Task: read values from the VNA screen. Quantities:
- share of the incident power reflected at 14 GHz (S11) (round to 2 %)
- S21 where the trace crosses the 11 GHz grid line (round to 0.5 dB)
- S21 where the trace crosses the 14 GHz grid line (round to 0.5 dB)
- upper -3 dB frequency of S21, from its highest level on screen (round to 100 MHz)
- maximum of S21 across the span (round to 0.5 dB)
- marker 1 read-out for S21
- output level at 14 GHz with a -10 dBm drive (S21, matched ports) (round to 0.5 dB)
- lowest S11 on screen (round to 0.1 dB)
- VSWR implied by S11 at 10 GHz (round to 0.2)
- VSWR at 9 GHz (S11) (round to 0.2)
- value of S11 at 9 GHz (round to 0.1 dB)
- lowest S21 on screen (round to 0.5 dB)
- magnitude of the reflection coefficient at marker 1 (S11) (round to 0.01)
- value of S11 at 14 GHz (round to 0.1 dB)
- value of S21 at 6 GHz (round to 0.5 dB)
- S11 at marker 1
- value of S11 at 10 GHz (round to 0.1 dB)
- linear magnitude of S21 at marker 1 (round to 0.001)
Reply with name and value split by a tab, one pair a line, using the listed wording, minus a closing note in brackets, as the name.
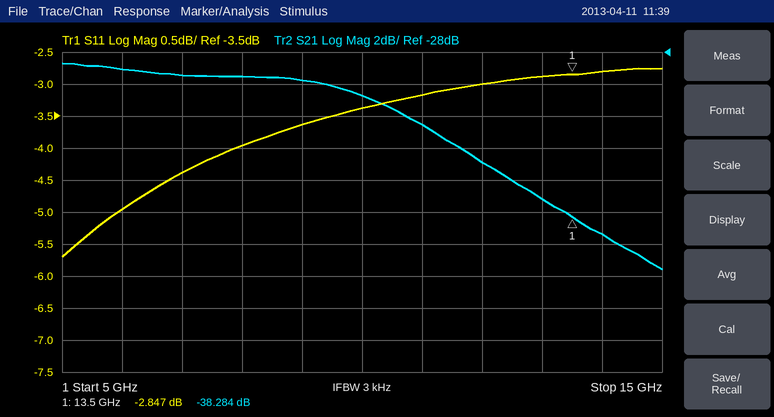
share of the incident power reflected at 14 GHz (S11)	52 %
S21 where the trace crosses the 11 GHz grid line	-32.5 dB
S21 where the trace crosses the 14 GHz grid line	-39.5 dB
upper -3 dB frequency of S21, from its highest level on screen	10.6 GHz
maximum of S21 across the span	-28.5 dB
marker 1 read-out for S21	-38.284 dB
output level at 14 GHz with a -10 dBm drive (S21, matched ports)	-49.5 dBm
lowest S11 on screen	-5.7 dB
VSWR implied by S11 at 10 GHz	5.2
VSWR at 9 GHz (S11)	4.8
value of S11 at 9 GHz	-3.6 dB
lowest S21 on screen	-41.5 dB
magnitude of the reflection coefficient at marker 1 (S11)	0.72
value of S11 at 14 GHz	-2.8 dB
value of S21 at 6 GHz	-29.0 dB
S11 at marker 1	-2.847 dB
value of S11 at 10 GHz	-3.4 dB
linear magnitude of S21 at marker 1	0.012
